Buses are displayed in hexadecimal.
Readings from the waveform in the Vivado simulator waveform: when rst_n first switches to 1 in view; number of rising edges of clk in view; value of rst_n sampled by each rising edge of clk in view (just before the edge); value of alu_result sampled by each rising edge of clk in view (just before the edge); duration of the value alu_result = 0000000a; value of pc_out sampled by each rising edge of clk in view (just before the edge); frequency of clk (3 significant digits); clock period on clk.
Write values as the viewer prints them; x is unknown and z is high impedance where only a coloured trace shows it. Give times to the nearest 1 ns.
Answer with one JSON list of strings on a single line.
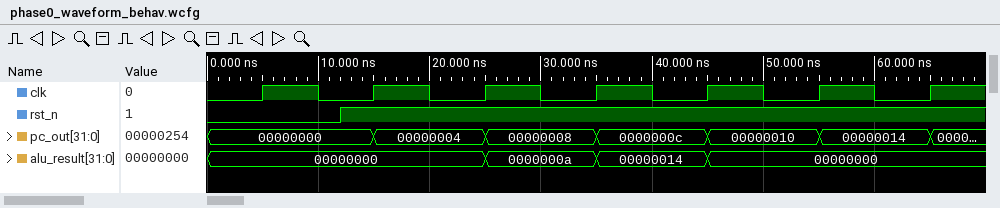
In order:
["12 ns", "7", "0 1 1 1 1 1 1", "00000000, 00000000, 00000000, 0000000a, 00000014, 00000000, 00000000", "10 ns", "00000000, 00000000, 00000004, 00000008, 0000000c, 00000010, 00000014", "100 MHz", "10 ns"]
